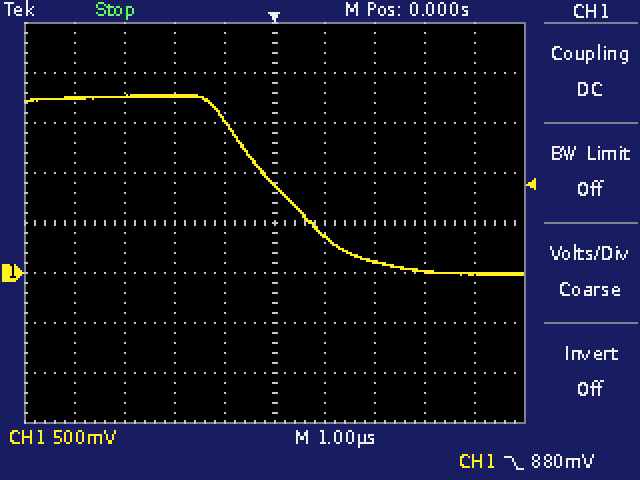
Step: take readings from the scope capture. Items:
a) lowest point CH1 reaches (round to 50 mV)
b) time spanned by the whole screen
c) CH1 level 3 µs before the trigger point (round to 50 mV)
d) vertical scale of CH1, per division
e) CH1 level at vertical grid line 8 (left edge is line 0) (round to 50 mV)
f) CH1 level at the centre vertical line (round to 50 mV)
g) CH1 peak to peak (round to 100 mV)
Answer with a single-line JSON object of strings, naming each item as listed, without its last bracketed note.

{"lowest point CH1 reaches": "0 mV", "time spanned by the whole screen": "10 µs", "CH1 level 3 µs before the trigger point": "1.75 V", "vertical scale of CH1, per division": "500 mV", "CH1 level at vertical grid line 8 (left edge is line 0)": "0 mV", "CH1 level at the centre vertical line": "900 mV", "CH1 peak to peak": "1.80 V"}
